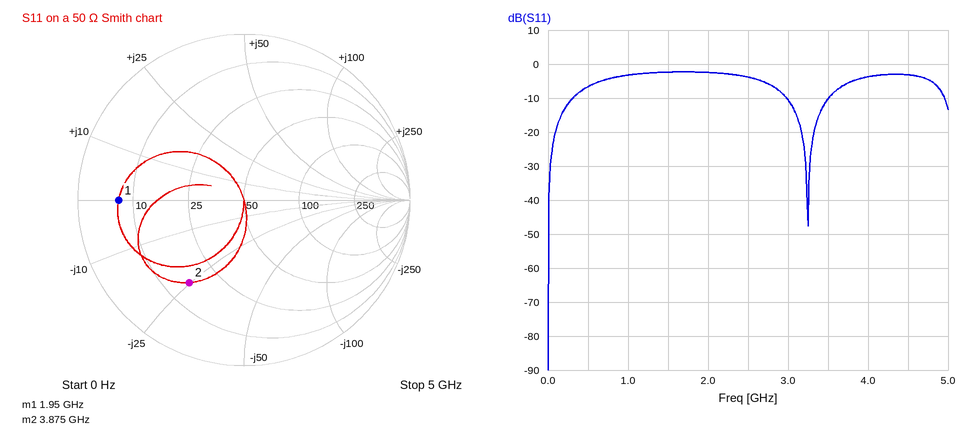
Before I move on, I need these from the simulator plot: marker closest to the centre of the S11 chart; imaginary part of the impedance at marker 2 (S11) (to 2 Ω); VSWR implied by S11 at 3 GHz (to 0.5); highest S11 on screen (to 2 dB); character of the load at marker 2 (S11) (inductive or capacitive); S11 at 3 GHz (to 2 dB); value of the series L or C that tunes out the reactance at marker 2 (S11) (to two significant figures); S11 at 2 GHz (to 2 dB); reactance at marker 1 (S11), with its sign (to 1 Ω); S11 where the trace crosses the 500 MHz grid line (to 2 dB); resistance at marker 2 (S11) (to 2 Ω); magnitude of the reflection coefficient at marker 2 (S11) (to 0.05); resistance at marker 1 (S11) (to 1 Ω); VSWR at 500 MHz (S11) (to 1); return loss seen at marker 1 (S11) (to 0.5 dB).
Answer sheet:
marker 2
-24 Ω
2.0
-2 dB
capacitive
-10 dB
1.0 nH
-2 dB
0 Ω
-6 dB
16 Ω
0.60
7 Ω
3
2.5 dB
